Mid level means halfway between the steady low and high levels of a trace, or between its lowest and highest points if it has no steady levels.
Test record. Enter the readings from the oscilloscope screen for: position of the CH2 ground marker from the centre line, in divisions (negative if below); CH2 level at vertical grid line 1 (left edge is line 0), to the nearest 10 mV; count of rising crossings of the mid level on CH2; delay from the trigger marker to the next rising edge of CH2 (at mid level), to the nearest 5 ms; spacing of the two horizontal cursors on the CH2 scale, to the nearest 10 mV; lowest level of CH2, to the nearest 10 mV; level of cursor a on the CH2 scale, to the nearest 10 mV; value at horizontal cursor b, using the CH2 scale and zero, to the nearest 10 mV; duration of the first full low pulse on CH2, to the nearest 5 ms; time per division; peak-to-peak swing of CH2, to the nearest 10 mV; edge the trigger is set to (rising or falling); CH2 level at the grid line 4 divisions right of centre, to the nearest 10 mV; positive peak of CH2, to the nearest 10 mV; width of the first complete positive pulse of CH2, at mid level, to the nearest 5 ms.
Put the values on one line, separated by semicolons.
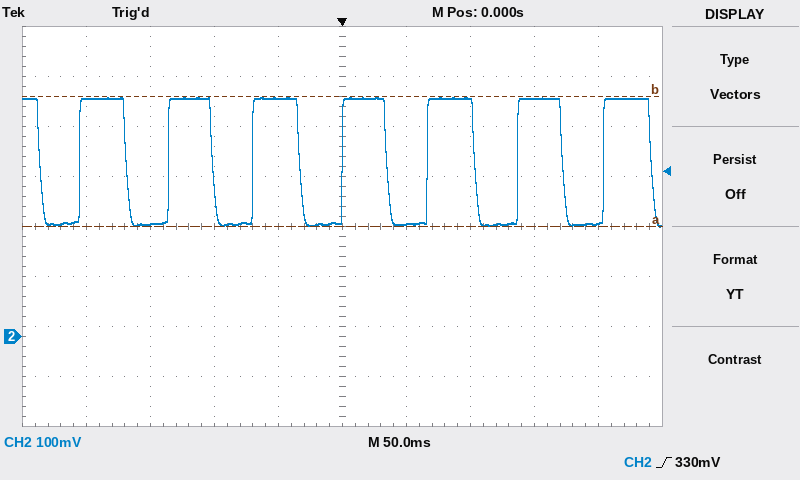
-2.2 div; 480 mV; 7; 65 ms; 260 mV; 220 mV; 220 mV; 480 mV; 30 ms; 50 ms; 260 mV; rising; 230 mV; 480 mV; 35 ms
